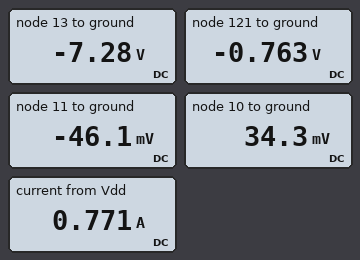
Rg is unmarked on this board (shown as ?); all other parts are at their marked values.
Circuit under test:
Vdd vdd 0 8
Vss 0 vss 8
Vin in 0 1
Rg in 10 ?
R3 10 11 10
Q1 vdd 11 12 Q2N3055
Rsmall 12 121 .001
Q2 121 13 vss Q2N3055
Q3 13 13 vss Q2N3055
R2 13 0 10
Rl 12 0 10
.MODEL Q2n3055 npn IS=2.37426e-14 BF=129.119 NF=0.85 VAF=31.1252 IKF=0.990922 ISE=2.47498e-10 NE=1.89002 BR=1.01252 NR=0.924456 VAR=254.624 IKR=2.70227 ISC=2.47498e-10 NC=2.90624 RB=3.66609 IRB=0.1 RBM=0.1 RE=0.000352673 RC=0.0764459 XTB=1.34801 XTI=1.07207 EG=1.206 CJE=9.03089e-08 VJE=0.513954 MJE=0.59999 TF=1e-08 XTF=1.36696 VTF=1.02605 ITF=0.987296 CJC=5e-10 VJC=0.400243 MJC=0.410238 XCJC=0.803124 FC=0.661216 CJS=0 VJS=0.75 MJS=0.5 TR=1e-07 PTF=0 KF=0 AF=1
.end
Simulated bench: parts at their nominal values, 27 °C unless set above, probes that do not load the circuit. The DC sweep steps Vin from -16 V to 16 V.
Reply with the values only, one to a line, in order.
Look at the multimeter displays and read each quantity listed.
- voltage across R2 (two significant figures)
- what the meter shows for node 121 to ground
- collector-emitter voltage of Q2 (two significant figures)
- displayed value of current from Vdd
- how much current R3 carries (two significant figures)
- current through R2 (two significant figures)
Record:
7.3 V
-0.763 V
7.2 V
0.771 A
8.0 mA
730 mA
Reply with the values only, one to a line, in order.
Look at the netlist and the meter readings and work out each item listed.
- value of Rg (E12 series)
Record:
120 Ω
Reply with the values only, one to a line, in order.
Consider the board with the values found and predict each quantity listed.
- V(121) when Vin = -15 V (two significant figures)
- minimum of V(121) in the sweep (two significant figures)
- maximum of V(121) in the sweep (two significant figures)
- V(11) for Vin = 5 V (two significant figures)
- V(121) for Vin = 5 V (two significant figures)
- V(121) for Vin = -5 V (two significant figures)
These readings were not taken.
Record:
-7.1 V
-7.1 V
7.8 V
3.0 V
2.2 V
-5.8 V
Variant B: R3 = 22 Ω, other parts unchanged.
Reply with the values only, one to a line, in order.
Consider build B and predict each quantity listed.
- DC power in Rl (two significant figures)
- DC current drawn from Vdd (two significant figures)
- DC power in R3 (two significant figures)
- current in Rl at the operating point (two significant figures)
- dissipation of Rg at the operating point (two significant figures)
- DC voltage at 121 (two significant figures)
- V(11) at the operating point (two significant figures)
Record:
70 mW
760 mA
1.4 mW
84 mA
7.5 mW
-840 mV
-120 mV
